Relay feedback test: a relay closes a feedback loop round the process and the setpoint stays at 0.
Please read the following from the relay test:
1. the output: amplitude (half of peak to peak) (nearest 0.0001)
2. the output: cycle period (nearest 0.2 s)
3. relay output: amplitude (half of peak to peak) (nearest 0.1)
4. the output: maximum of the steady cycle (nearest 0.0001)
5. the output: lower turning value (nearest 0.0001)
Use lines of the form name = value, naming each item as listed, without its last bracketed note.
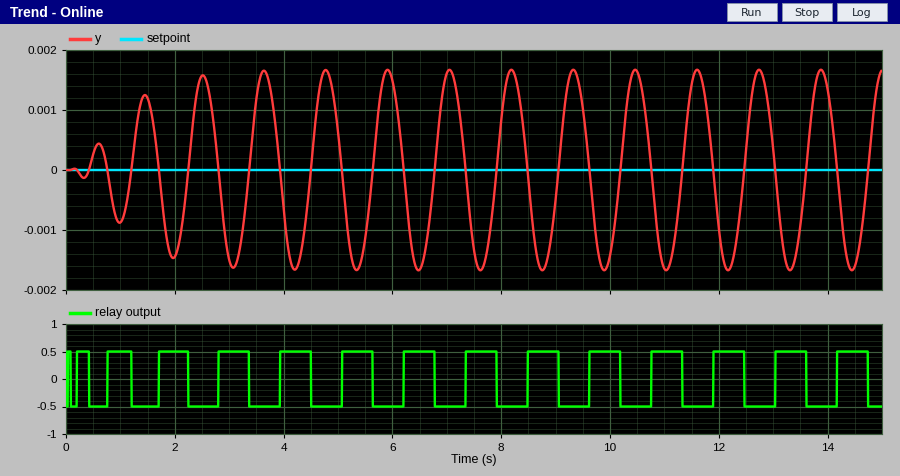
the output: amplitude (half of peak to peak) = 0.0017
the output: cycle period = 1.2 s
relay output: amplitude (half of peak to peak) = 0.5
the output: maximum of the steady cycle = 0.0017
the output: lower turning value = -0.0017
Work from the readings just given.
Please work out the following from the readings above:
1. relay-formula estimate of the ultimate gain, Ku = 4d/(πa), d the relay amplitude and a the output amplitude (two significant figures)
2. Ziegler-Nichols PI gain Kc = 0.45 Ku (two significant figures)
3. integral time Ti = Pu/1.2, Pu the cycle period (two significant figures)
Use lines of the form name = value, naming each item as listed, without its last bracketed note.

relay-formula estimate of the ultimate gain, Ku = 4d/(πa), d the relay amplitude and a the output amplitude = 370
Ziegler-Nichols PI gain Kc = 0.45 Ku = 170
integral time Ti = Pu/1.2, Pu the cycle period = 1.0 s
